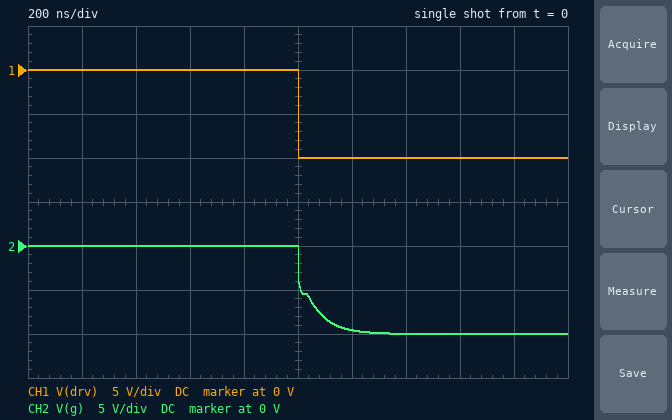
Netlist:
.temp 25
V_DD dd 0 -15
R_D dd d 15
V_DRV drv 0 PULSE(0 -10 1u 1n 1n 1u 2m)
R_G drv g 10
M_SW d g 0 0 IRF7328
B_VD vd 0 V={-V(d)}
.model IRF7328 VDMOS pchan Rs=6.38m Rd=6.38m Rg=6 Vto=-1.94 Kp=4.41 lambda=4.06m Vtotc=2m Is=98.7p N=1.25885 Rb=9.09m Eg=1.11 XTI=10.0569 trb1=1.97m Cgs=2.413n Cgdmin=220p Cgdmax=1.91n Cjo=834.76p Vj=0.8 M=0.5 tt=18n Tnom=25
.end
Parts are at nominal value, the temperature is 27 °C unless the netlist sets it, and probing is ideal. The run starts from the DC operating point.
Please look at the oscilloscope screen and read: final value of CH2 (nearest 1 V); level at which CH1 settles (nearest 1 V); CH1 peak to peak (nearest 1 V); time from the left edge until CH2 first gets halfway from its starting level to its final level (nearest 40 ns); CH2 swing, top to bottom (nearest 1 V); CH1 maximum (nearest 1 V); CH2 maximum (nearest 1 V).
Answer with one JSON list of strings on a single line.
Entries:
["-10 V", "-10 V", "10 V", "1.00 µs", "10 V", "0 V", "0 V"]
